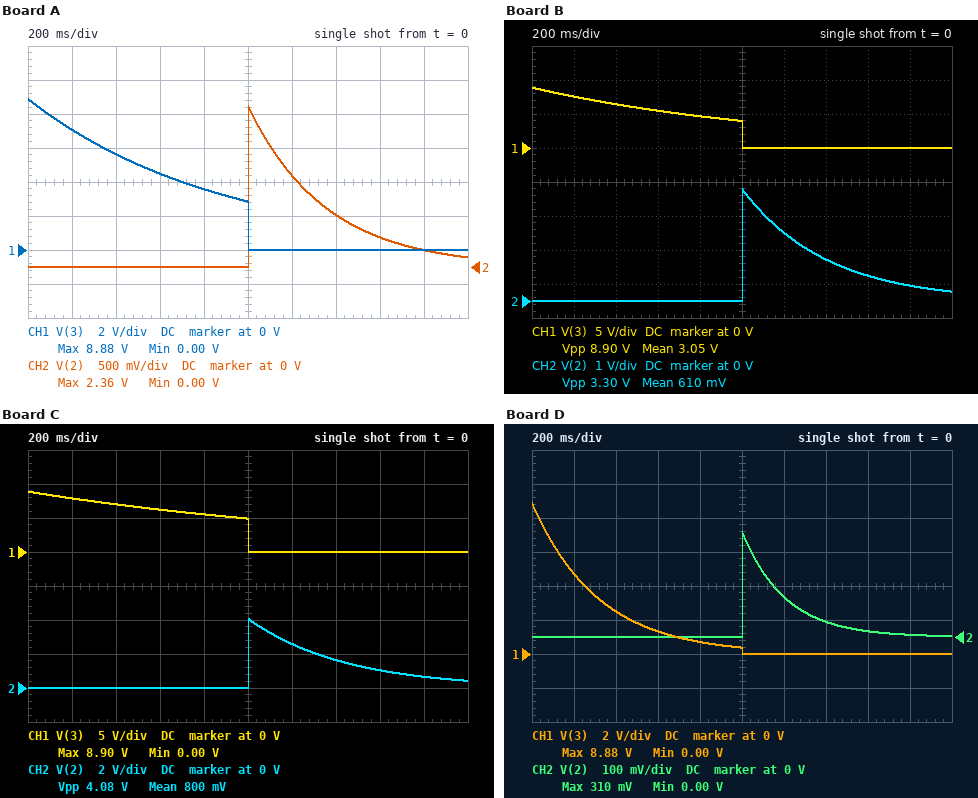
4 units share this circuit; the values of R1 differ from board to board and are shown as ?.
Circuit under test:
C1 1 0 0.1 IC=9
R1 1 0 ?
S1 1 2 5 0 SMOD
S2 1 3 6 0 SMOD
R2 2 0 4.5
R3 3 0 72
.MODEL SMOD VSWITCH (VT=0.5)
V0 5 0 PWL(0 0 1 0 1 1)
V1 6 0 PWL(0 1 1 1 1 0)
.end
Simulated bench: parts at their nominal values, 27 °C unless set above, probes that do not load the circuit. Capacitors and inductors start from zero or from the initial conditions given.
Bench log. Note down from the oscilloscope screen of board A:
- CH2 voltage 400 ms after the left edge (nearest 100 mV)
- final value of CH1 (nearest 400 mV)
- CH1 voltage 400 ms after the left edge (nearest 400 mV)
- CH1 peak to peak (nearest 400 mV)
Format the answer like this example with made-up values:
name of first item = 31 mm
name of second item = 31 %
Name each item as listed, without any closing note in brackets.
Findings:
CH2 voltage 400 ms after the left edge = 0 V
final value of CH1 = 0 V
CH1 voltage 400 ms after the left edge = 5.6 V
CH1 peak to peak = 8.8 V
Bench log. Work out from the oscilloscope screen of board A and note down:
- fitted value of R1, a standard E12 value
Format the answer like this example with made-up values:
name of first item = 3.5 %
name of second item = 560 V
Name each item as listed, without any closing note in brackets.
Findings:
fitted value of R1, a standard E12 value = 10 Ω
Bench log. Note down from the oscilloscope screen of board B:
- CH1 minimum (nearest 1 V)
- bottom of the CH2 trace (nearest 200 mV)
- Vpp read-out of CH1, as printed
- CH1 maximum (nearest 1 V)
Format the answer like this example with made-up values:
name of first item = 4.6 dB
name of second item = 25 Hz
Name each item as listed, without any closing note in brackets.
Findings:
CH1 minimum = 0 V
bottom of the CH2 trace = 0 V
Vpp read-out of CH1, as printed = 8.90 V
CH1 maximum = 9 V
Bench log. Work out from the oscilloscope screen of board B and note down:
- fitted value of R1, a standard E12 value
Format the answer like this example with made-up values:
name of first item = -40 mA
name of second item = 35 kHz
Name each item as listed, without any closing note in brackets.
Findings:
fitted value of R1, a standard E12 value = 15 Ω
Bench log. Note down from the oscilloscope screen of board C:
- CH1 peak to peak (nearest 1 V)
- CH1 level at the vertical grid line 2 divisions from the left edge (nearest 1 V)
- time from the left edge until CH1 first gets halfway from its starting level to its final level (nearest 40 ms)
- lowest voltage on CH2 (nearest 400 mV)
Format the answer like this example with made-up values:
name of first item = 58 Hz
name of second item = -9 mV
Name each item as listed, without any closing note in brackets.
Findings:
CH1 peak to peak = 9 V
CH1 level at the vertical grid line 2 divisions from the left edge = 7 V
time from the left edge until CH1 first gets halfway from its starting level to its final level = 1.00 s
lowest voltage on CH2 = 0 V
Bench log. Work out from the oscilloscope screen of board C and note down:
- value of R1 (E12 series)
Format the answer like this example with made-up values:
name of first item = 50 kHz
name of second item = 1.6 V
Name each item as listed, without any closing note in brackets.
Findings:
value of R1 = 22 Ω
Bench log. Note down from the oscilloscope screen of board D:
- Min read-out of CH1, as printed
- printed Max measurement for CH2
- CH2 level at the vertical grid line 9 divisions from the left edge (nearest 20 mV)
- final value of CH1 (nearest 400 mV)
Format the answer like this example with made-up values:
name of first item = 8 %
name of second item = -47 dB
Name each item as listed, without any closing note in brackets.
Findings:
Min read-out of CH1, as printed = 0.00 V
printed Max measurement for CH2 = 310 mV
CH2 level at the vertical grid line 9 divisions from the left edge = 0 V
final value of CH1 = 0 V
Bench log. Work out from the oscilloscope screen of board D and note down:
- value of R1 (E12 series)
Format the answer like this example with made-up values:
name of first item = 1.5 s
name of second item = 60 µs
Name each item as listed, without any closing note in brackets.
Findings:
value of R1 = 3.3 Ω
